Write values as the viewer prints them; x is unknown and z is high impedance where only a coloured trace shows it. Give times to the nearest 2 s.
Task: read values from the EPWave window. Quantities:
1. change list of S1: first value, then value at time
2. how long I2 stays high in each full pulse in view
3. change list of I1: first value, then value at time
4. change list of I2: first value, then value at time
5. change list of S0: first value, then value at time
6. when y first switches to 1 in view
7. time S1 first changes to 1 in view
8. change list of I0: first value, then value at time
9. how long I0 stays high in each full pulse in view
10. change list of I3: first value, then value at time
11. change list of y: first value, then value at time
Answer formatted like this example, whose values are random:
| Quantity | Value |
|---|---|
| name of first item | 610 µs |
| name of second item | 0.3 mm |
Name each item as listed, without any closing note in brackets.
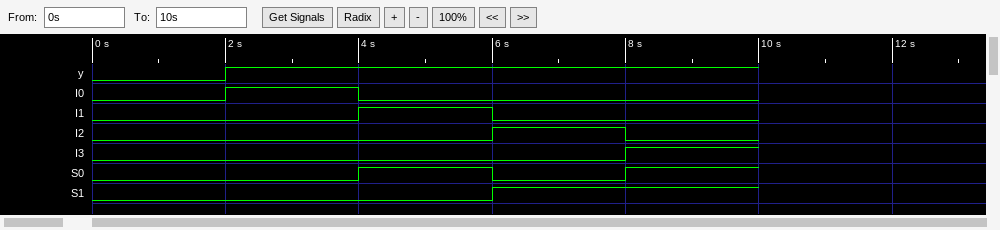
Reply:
| Quantity | Value |
|---|---|
| change list of S1: first value, then value at time | 0, 1 at 6 s |
| how long I2 stays high in each full pulse in view | 2 s |
| change list of I1: first value, then value at time | 0, 1 at 4 s, 0 at 6 s |
| change list of I2: first value, then value at time | 0, 1 at 6 s, 0 at 8 s |
| change list of S0: first value, then value at time | 0, 1 at 4 s, 0 at 6 s, 1 at 8 s |
| when y first switches to 1 in view | 2 s |
| time S1 first changes to 1 in view | 6 s |
| change list of I0: first value, then value at time | 0, 1 at 2 s, 0 at 4 s |
| how long I0 stays high in each full pulse in view | 2 s |
| change list of I3: first value, then value at time | 0, 1 at 8 s |
| change list of y: first value, then value at time | 0, 1 at 2 s |
